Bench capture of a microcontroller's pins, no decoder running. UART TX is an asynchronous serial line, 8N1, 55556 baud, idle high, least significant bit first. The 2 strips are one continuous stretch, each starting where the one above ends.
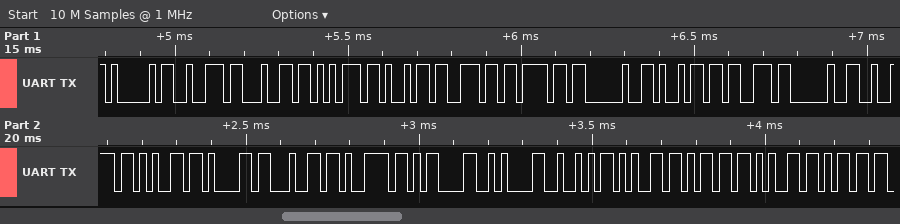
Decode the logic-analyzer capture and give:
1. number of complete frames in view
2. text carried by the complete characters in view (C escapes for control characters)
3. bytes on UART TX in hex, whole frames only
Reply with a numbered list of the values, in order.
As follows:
1. 23
2. "Arduino is ready\r\nRemem"
3. 41 72 64 75 69 6E 6F 20 69 73 20 72 65 61 64 79 0D 0A 52 65 6D 65 6D
